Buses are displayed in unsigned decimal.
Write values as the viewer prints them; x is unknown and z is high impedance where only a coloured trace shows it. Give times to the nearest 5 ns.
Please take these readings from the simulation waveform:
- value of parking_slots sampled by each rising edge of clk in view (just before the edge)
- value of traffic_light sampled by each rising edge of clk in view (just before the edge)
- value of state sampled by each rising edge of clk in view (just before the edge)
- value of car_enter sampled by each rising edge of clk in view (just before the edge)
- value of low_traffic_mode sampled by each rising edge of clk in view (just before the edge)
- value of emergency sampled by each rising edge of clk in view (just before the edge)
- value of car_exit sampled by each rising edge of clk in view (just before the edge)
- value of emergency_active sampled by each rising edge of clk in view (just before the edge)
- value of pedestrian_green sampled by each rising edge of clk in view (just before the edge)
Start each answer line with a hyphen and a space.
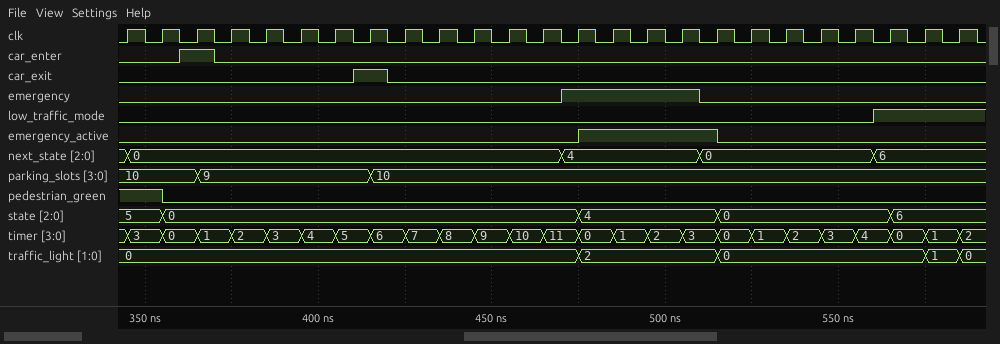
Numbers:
- 10, 10, 10, 9, 9, 9, 9, 9, 10, 10, 10, 10, 10, 10, 10, 10, 10, 10, 10, 10, 10, 10, 10, 10, 10
- 0, 0, 0, 0, 0, 0, 0, 0, 0, 0, 0, 0, 0, 0, 2, 2, 2, 2, 0, 0, 0, 0, 0, 0, 1
- 5, 5, 0, 0, 0, 0, 0, 0, 0, 0, 0, 0, 0, 0, 4, 4, 4, 4, 0, 0, 0, 0, 0, 6, 6
- 0 0 1 0 0 0 0 0 0 0 0 0 0 0 0 0 0 0 0 0 0 0 0 0 0
- 0 0 0 0 0 0 0 0 0 0 0 0 0 0 0 0 0 0 0 0 0 0 1 1 1
- 0 0 0 0 0 0 0 0 0 0 0 0 0 1 1 1 1 0 0 0 0 0 0 0 0
- 0 0 0 0 0 0 0 1 0 0 0 0 0 0 0 0 0 0 0 0 0 0 0 0 0
- 0 0 0 0 0 0 0 0 0 0 0 0 0 0 1 1 1 1 0 0 0 0 0 0 0
- 1 1 0 0 0 0 0 0 0 0 0 0 0 0 0 0 0 0 0 0 0 0 0 0 0
